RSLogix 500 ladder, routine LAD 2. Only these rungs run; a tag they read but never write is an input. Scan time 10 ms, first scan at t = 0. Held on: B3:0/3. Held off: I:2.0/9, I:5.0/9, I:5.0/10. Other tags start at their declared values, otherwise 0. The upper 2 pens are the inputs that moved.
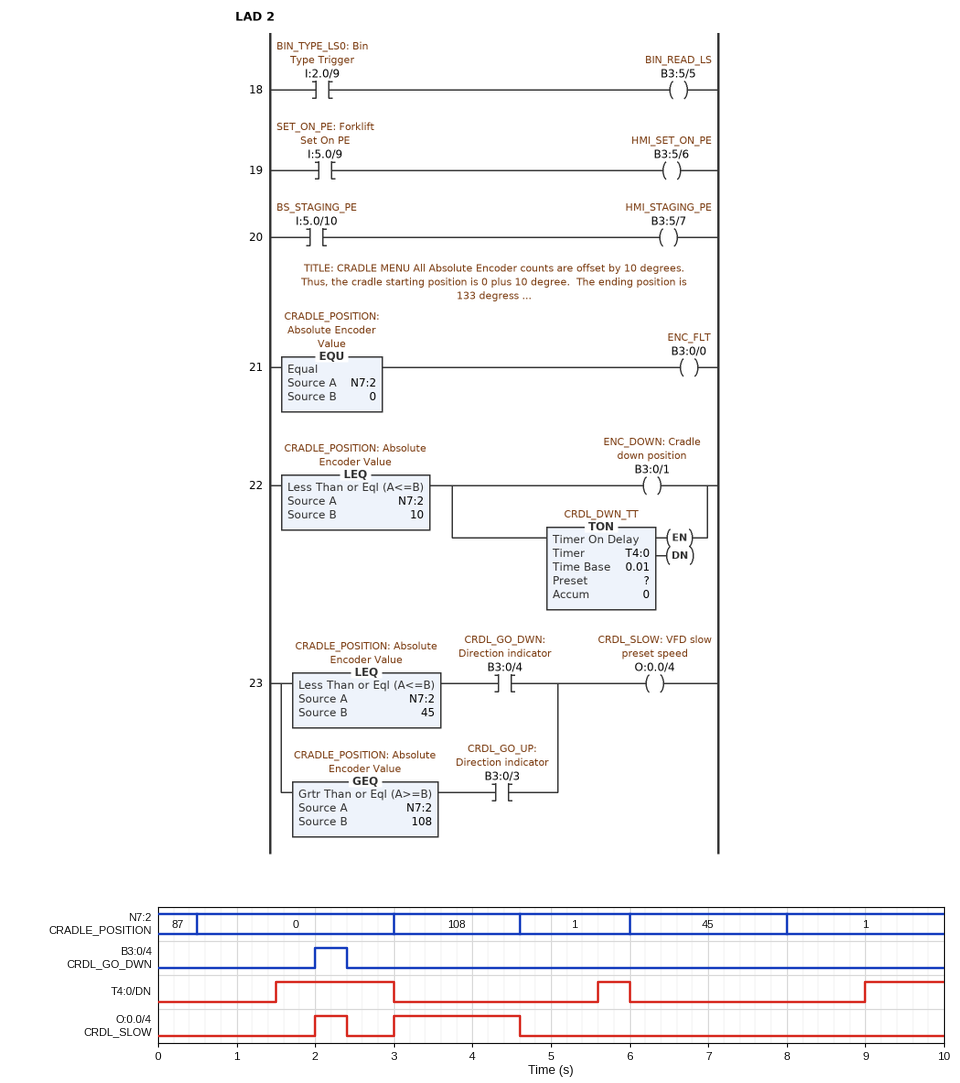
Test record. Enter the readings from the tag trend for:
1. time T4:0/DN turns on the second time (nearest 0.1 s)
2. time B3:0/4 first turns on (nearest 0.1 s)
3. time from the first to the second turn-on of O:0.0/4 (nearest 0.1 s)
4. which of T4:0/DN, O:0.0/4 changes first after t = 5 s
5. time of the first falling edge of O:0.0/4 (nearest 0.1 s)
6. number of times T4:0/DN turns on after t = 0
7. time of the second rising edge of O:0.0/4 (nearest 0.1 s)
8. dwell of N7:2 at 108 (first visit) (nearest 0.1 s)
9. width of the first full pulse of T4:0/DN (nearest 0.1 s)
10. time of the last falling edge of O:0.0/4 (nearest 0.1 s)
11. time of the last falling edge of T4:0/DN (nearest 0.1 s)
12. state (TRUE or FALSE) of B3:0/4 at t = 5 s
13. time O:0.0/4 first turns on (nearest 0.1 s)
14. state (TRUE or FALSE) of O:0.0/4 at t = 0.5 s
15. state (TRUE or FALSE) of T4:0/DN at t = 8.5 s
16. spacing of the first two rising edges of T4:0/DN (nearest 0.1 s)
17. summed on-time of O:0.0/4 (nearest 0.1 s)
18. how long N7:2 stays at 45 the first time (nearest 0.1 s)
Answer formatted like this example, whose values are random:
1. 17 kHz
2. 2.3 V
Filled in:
1. 5.6 s
2. 2.0 s
3. 1.0 s
4. T4:0/DN
5. 2.4 s
6. 3
7. 3.0 s
8. 1.6 s
9. 1.5 s
10. 4.6 s
11. 6.0 s
12. FALSE
13. 2.0 s
14. FALSE
15. FALSE
16. 4.1 s
17. 2.0 s
18. 2.0 s
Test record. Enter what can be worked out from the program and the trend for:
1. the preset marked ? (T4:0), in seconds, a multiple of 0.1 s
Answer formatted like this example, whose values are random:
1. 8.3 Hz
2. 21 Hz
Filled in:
1. 1.0 s
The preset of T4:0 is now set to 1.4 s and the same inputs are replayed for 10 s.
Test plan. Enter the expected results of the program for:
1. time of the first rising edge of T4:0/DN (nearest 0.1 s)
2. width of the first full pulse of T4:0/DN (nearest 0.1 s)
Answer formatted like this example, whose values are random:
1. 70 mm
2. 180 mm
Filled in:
1. 1.9 s
2. 1.1 s
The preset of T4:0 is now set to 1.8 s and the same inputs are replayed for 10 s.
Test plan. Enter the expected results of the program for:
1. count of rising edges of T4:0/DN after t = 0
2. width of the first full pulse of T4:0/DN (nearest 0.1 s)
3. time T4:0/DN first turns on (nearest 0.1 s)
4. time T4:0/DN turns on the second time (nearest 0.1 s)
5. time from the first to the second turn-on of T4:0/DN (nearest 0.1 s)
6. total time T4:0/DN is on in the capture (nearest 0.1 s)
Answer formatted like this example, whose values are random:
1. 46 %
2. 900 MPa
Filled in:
1. 2
2. 0.7 s
3. 2.3 s
4. 9.8 s
5. 7.5 s
6. 0.9 s
